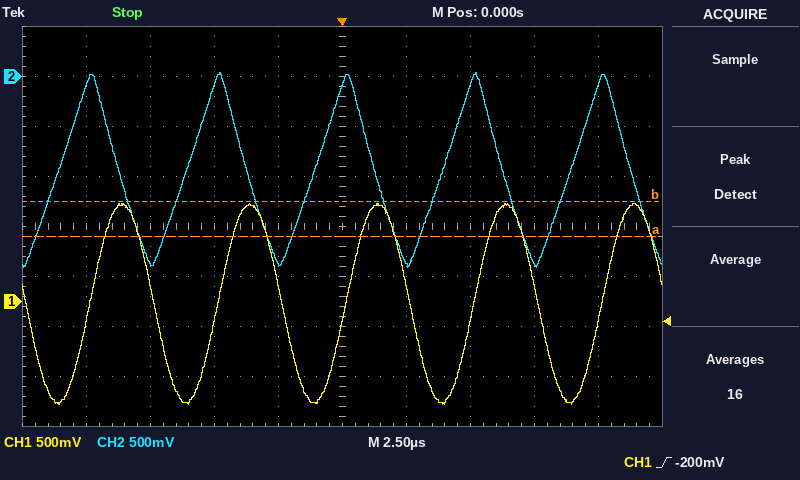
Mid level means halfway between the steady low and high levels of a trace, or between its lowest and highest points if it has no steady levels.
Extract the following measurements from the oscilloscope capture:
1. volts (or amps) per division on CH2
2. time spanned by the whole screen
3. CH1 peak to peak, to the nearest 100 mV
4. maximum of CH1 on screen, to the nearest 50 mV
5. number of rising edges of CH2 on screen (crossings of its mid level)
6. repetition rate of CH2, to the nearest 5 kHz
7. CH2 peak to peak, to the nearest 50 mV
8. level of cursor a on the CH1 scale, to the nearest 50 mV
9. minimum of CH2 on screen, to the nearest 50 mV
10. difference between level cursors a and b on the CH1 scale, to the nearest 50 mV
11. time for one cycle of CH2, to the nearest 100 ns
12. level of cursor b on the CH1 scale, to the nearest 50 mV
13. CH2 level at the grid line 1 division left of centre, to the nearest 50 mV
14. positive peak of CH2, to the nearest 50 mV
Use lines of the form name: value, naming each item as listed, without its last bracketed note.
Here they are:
volts (or amps) per division on CH2: 500 mV
time spanned by the whole screen: 25 µs
CH1 peak to peak, to the nearest 100 mV: 2.00 V
maximum of CH1 on screen, to the nearest 50 mV: 1.00 V
number of rising edges of CH2 on screen: 5
repetition rate of CH2, to the nearest 5 kHz: 200 kHz
CH2 peak to peak, to the nearest 50 mV: 1.95 V
level of cursor a on the CH1 scale, to the nearest 50 mV: 650 mV
minimum of CH2 on screen, to the nearest 50 mV: -1.90 V
difference between level cursors a and b on the CH1 scale, to the nearest 50 mV: 350 mV
time for one cycle of CH2, to the nearest 100 ns: 5.0 µs
level of cursor b on the CH1 scale, to the nearest 50 mV: 1.00 V
CH2 level at the grid line 1 division left of centre, to the nearest 50 mV: -1.85 V
positive peak of CH2, to the nearest 50 mV: 50 mV
